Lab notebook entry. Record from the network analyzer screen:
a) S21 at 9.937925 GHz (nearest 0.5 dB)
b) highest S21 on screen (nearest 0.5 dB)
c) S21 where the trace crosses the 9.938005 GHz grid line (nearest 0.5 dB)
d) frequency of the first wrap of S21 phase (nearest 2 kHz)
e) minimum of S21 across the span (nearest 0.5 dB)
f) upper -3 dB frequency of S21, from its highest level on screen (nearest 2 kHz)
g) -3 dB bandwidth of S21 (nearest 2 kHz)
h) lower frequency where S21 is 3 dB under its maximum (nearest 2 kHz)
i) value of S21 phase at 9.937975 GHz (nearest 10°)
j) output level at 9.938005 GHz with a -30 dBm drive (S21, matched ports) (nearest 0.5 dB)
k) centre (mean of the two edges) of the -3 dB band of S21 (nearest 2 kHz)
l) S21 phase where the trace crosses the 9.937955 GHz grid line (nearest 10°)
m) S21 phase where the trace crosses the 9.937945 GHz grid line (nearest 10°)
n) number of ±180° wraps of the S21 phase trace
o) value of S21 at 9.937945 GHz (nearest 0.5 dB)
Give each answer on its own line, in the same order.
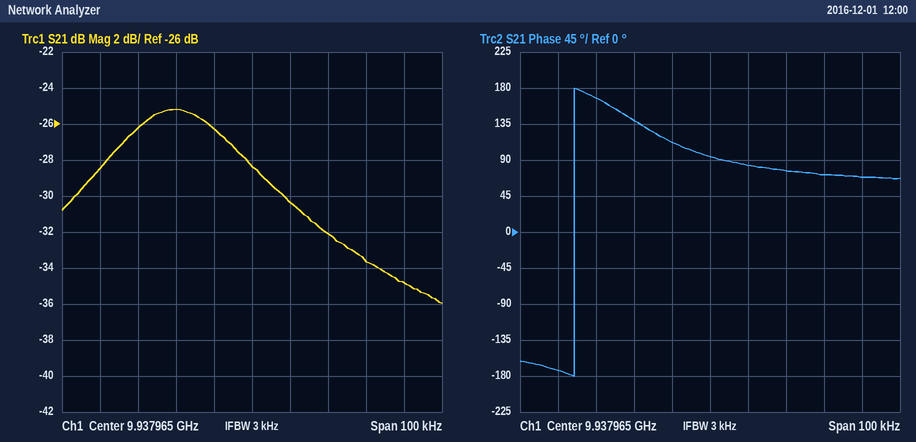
-28.5 dB
-25.0 dB
-35.0 dB
9.937930 GHz
-36.0 dB
9.937964 GHz
38 kHz
9.937926 GHz
80°
-65.0 dBm
9.937946 GHz
110°
140°
1
-25.0 dB
